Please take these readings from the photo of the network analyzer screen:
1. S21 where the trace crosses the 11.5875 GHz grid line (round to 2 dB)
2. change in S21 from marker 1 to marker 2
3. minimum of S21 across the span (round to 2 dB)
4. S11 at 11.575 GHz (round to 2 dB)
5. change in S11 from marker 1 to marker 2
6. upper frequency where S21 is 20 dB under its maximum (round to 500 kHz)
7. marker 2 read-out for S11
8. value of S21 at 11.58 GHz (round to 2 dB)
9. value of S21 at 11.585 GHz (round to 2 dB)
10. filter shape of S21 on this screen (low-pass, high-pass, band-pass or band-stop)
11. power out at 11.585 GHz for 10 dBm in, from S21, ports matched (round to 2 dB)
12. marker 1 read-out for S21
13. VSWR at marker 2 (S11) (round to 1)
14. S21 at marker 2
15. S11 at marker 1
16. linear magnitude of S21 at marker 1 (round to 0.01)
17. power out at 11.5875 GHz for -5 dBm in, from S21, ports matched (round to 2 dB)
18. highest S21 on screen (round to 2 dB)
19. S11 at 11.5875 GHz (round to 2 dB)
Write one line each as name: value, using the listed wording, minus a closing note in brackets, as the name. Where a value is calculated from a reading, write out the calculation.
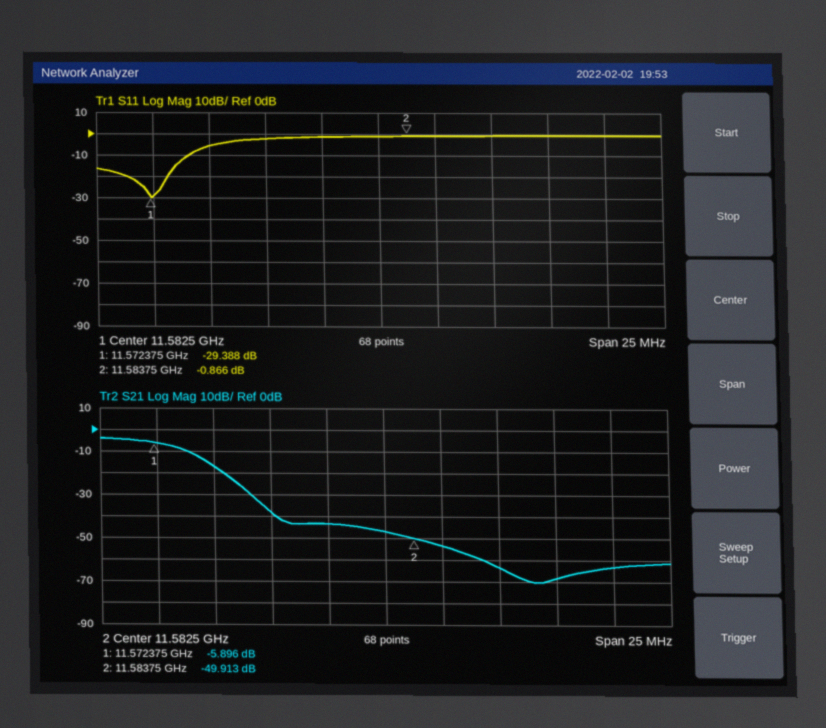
S21 where the trace crosses the 11.5875 GHz grid line: -64 dB
change in S21 from marker 1 to marker 2: -49.913 − (-5.896) = -44.017 dB
minimum of S21 across the span: -70 dB
S11 at 11.575 GHz: -6 dB
change in S11 from marker 1 to marker 2: -0.866 − (-29.388) = 28.522 dB
upper frequency where S21 is 20 dB under its maximum: 11.5760 GHz
marker 2 read-out for S11: -0.866 dB
value of S21 at 11.58 GHz: -44 dB
value of S21 at 11.585 GHz: -54 dB
filter shape of S21 on this screen: low-pass
power out at 11.585 GHz for 10 dBm in, from S21, ports matched: 10 dBm + (-54 dB) = -44 dBm
marker 1 read-out for S21: -5.896 dB
VSWR at marker 2 (S11): (1 + 0.9051)/(1 − 0.9051) ≈ 20
S21 at marker 2: -49.913 dB
S11 at marker 1: -29.388 dB
linear magnitude of S21 at marker 1: 10^(-5.896/20) ≈ 0.51
power out at 11.5875 GHz for -5 dBm in, from S21, ports matched: -5 dBm + (-64 dB) = -68 dBm
highest S21 on screen: -4 dB
S11 at 11.5875 GHz: 0 dB
